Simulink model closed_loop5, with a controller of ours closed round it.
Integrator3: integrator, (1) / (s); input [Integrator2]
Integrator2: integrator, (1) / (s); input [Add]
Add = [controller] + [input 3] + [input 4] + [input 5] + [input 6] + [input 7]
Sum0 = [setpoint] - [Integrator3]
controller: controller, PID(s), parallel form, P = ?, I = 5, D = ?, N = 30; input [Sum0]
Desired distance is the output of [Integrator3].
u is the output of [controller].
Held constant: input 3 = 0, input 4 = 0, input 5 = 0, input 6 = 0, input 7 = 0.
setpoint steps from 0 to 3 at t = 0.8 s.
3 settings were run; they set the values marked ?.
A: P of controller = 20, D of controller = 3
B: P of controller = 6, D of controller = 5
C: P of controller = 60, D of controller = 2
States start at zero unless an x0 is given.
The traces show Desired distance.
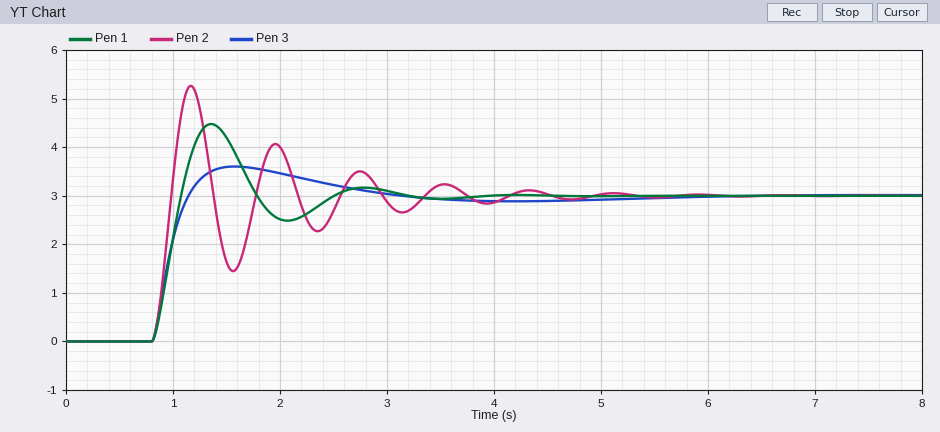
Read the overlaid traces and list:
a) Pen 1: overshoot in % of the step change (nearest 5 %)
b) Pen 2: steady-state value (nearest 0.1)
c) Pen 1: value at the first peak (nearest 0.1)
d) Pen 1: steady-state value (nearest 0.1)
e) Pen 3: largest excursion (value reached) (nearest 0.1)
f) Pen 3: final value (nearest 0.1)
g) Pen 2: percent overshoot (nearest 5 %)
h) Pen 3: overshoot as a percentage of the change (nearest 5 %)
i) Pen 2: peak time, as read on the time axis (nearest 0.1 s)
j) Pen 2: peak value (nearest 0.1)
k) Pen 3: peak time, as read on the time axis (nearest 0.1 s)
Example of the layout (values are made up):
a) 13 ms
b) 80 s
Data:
a) 50 %
b) 3.0
c) 4.5
d) 3.0
e) 3.6
f) 3.0
g) 75 %
h) 20 %
i) 1.2 s
j) 5.3
k) 1.6 s
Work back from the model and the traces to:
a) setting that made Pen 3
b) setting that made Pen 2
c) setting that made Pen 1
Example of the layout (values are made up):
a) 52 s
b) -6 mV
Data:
a) B
b) C
c) A
